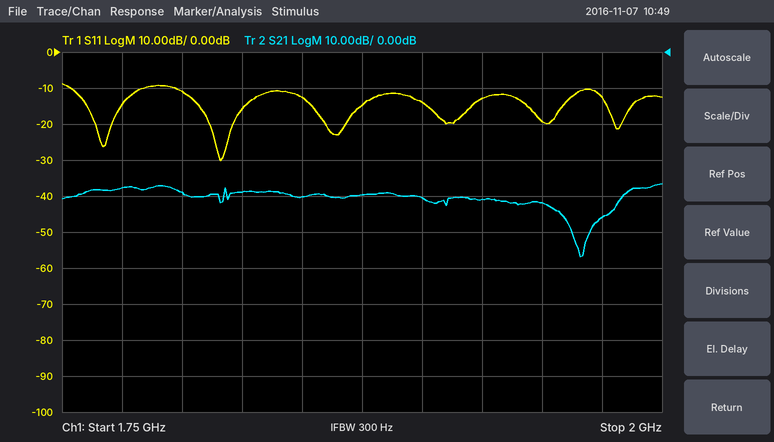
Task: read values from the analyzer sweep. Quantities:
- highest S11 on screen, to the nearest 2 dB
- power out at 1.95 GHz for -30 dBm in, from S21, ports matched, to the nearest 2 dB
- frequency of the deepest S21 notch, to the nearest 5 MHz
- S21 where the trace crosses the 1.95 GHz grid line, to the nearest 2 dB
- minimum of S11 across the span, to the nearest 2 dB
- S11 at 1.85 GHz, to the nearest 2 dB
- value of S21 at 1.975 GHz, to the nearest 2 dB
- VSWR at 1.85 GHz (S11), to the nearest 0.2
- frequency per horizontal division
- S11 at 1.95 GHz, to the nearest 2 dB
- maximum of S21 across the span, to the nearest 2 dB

-8 dB
-72 dBm
1.965 GHz
-42 dB
-30 dB
-12 dB
-46 dB
1.6
25 MHz
-20 dB
-36 dB
